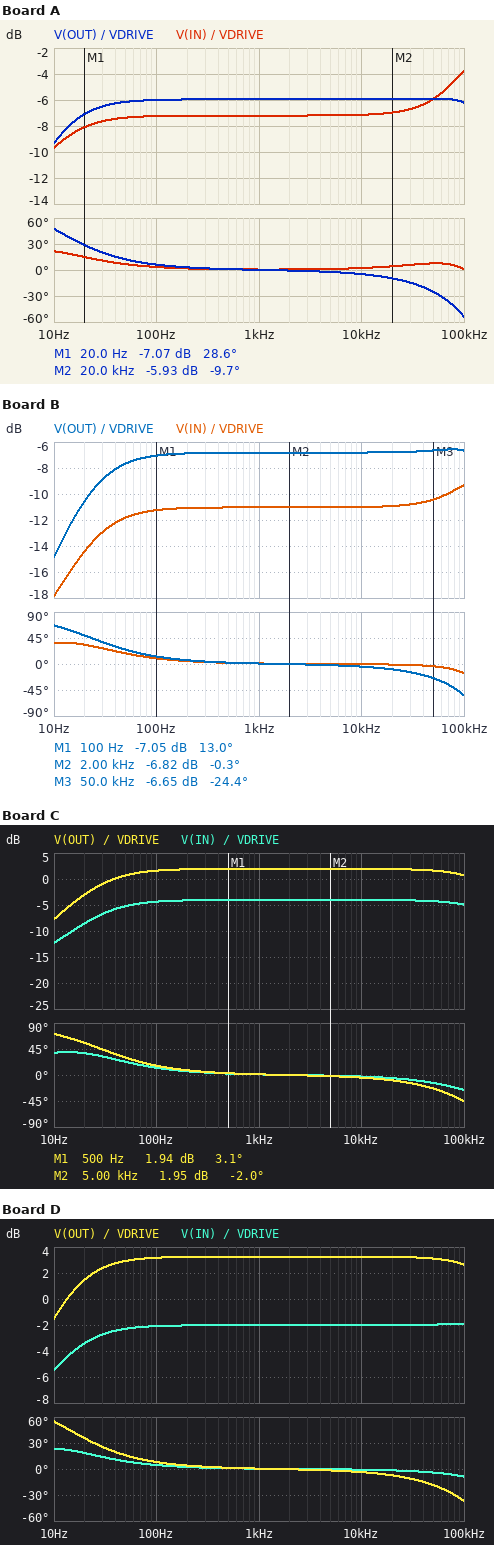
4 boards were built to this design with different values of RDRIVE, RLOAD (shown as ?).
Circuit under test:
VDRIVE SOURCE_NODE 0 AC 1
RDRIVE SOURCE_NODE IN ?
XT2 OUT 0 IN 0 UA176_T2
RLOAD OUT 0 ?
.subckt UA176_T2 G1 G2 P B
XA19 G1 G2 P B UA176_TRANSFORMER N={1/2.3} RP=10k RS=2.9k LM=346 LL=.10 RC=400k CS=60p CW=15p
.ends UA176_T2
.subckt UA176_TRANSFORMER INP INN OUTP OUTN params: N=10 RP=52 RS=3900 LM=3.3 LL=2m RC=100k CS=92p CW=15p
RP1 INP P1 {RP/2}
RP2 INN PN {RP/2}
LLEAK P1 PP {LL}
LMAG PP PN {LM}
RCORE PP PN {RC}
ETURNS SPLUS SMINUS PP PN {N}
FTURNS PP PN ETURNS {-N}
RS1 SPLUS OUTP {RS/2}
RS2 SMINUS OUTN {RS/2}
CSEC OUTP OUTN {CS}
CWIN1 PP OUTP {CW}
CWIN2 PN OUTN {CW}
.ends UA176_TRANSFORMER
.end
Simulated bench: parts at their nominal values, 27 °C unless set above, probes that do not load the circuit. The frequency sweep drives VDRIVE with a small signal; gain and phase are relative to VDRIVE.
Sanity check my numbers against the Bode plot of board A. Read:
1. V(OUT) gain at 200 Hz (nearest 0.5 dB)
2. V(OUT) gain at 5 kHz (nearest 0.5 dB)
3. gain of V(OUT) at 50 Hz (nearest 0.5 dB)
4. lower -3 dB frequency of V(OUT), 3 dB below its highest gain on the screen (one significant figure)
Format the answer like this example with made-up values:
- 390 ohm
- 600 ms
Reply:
- -6.0 dB
- -6.0 dB
- -6.0 dB
- 10 Hz
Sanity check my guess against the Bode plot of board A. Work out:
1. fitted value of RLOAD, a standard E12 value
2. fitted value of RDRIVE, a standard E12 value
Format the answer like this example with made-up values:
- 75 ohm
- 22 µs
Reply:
- 27 kΩ
- 12 kΩ
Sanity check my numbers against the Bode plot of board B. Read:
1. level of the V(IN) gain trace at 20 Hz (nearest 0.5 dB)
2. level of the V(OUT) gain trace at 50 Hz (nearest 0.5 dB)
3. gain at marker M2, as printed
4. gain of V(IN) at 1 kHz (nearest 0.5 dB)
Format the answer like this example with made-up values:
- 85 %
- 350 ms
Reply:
- -14.5 dB
- -7.5 dB
- -6.82 dB
- -11.0 dB
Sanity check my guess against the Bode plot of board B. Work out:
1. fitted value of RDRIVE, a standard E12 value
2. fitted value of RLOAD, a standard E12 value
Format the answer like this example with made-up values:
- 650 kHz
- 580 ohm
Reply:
- 39 kΩ
- 68 kΩ
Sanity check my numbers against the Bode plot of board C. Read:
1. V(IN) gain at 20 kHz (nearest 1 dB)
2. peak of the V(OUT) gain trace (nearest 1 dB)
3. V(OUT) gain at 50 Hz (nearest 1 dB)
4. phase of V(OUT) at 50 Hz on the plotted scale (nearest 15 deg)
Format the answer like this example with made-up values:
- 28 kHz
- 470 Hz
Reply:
- -4 dB
- 2 dB
- 1 dB
- 30 deg
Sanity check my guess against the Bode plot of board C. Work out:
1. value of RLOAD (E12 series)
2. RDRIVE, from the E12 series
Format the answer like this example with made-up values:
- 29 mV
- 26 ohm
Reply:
- 220 kΩ
- 18 kΩ
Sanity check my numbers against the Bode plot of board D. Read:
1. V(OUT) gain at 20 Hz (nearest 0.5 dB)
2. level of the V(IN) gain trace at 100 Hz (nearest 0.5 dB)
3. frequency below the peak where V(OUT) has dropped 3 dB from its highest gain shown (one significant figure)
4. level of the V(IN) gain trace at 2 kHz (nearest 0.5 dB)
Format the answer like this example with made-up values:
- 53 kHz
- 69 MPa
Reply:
- 1.5 dB
- -2.0 dB
- 10 Hz
- -2.0 dB
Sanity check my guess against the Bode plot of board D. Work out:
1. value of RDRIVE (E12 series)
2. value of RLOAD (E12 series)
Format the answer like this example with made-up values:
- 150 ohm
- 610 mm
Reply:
- 5.6 kΩ
- 120 kΩ
